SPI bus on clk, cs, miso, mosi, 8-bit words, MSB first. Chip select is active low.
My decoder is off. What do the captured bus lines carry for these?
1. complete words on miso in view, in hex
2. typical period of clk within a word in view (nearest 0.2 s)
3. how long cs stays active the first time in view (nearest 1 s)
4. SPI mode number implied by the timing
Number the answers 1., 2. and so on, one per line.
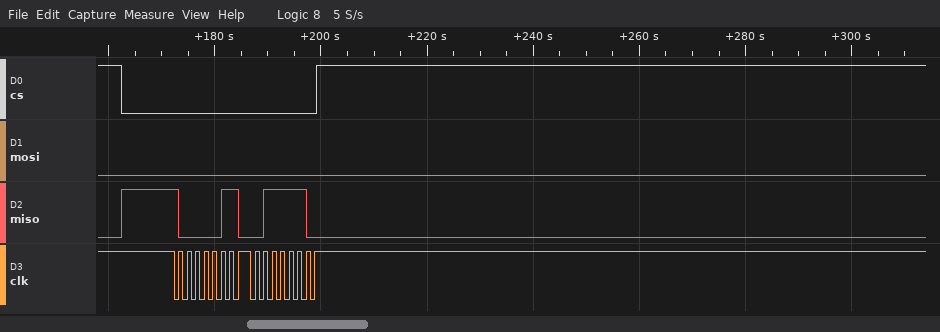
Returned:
1. 83, 3E
2. 1.6 s
3. 37 s
4. 2
